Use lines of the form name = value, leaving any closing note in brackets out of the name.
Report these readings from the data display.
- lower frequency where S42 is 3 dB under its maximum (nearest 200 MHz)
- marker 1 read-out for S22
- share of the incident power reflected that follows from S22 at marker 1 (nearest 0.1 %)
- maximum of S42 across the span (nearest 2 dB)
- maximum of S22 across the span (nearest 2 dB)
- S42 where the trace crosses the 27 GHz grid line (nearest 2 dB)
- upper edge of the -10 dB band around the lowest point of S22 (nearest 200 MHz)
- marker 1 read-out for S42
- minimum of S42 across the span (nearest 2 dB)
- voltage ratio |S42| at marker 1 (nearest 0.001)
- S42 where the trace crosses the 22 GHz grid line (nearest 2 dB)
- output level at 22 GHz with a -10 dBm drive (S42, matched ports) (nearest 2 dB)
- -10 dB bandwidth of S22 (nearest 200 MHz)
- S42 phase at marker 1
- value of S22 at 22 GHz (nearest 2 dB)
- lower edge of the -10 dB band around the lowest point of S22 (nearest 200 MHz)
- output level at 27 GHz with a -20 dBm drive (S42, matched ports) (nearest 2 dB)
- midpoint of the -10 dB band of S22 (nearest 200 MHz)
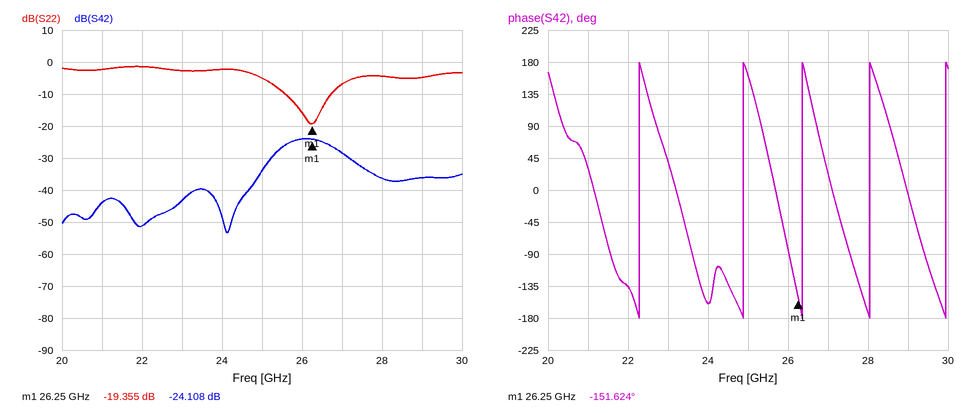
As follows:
lower frequency where S42 is 3 dB under its maximum = 25.4 GHz
marker 1 read-out for S22 = -19.355 dB
share of the incident power reflected that follows from S22 at marker 1 = 1.2 %
maximum of S42 across the span = -24 dB
maximum of S22 across the span = -2 dB
S42 where the trace crosses the 27 GHz grid line = -28 dB
upper edge of the -10 dB band around the lowest point of S22 = 26.8 GHz
marker 1 read-out for S42 = -24.108 dB
minimum of S42 across the span = -54 dB
voltage ratio |S42| at marker 1 = 0.062
S42 where the trace crosses the 22 GHz grid line = -52 dB
output level at 22 GHz with a -10 dBm drive (S42, matched ports) = -62 dBm
-10 dB bandwidth of S22 = 1.2 GHz
S42 phase at marker 1 = -151.624°
value of S22 at 22 GHz = -2 dB
lower edge of the -10 dB band around the lowest point of S22 = 25.6 GHz
output level at 27 GHz with a -20 dBm drive (S42, matched ports) = -48 dBm
midpoint of the -10 dB band of S22 = 26.2 GHz
